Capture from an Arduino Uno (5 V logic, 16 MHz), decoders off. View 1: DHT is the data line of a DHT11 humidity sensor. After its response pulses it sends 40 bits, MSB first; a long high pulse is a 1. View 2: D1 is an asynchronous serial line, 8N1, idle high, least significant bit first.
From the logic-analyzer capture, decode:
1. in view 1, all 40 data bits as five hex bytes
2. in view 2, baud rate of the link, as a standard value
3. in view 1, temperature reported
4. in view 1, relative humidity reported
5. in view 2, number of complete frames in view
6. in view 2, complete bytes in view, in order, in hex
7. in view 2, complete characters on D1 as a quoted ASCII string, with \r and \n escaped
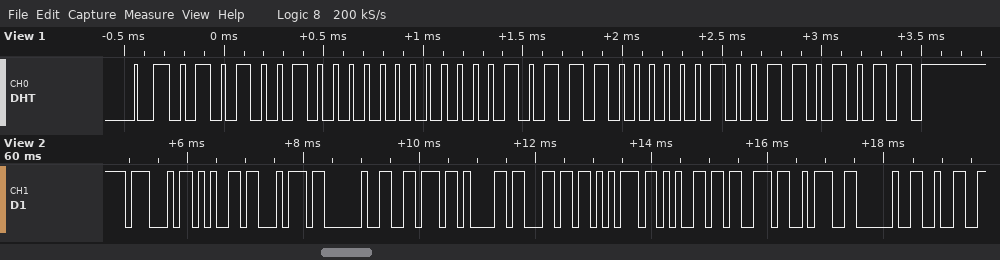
52 00 17 02 6B
9600 baud
23.2 °C
82 %
13
0x47 0x65 0x74 0x20 0x76 0x61 0x6C 0x75 0x65 0x73 0x3A 0x20 0x32
"Get values: 2"
